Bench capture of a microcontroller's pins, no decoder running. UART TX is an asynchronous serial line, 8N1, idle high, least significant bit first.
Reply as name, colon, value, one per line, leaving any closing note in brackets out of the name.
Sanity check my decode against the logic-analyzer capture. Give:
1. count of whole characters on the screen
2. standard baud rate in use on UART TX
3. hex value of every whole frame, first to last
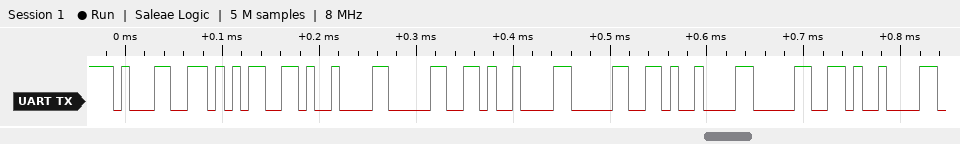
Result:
count of whole characters on the screen: 9
standard baud rate in use on UART TX: 115200 baud
hex value of every whole frame, first to last: 0x31 0x35 0x09 0x30 0x09 0x30 0x09 0x30 0x09
